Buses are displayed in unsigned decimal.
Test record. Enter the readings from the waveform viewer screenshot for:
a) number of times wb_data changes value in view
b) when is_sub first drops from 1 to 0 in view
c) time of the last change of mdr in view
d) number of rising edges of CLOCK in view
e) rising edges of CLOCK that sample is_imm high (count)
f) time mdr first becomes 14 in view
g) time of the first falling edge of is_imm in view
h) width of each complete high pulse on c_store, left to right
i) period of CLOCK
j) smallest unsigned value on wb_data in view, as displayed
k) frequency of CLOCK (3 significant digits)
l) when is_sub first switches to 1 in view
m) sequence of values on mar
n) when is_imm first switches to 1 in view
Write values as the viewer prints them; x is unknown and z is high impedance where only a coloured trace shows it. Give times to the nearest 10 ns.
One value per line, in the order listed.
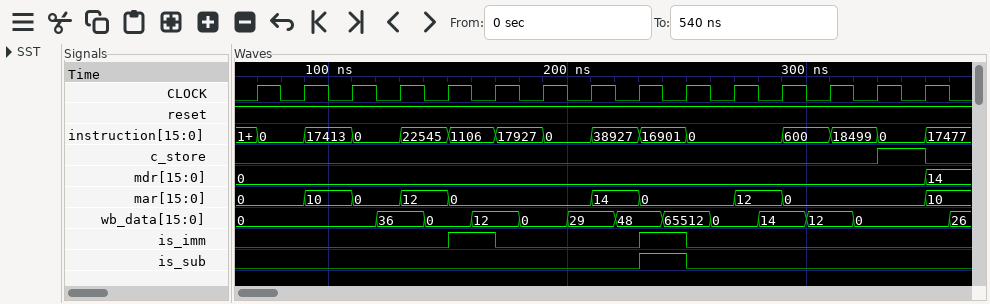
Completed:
12
250 ns
350 ns
15
2
350 ns
170 ns
20 ns
20 ns
0
50.0 MHz
230 ns
0, 10, 0, 12, 0, 14, 0, 12, 0, 10
150 ns
